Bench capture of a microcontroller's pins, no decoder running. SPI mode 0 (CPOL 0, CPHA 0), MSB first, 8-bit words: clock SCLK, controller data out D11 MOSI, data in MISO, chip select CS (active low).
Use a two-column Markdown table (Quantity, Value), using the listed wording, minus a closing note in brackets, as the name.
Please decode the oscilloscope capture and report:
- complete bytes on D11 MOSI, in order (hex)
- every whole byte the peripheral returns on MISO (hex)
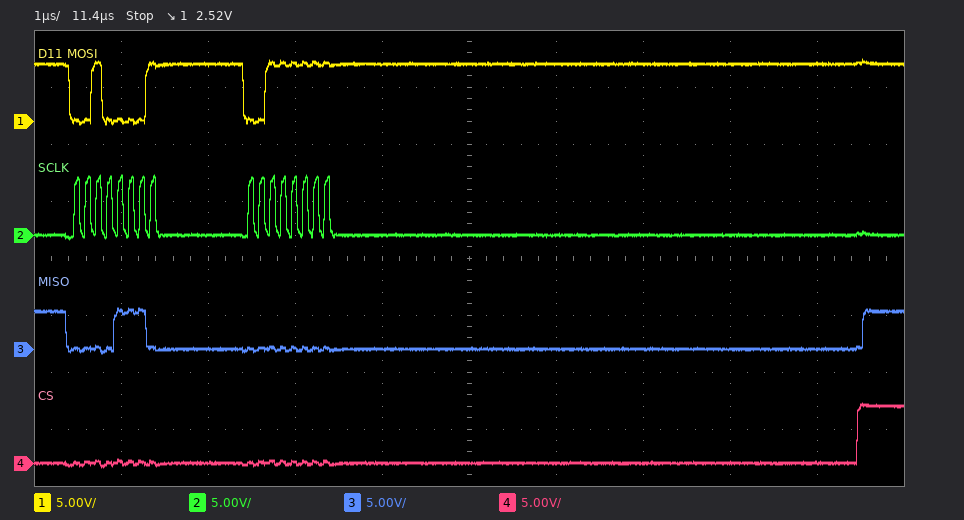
| Quantity | Value |
|---|---|
| complete bytes on D11 MOSI, in order | 21 3F |
| every whole byte the peripheral returns on MISO | 0E 00 |
